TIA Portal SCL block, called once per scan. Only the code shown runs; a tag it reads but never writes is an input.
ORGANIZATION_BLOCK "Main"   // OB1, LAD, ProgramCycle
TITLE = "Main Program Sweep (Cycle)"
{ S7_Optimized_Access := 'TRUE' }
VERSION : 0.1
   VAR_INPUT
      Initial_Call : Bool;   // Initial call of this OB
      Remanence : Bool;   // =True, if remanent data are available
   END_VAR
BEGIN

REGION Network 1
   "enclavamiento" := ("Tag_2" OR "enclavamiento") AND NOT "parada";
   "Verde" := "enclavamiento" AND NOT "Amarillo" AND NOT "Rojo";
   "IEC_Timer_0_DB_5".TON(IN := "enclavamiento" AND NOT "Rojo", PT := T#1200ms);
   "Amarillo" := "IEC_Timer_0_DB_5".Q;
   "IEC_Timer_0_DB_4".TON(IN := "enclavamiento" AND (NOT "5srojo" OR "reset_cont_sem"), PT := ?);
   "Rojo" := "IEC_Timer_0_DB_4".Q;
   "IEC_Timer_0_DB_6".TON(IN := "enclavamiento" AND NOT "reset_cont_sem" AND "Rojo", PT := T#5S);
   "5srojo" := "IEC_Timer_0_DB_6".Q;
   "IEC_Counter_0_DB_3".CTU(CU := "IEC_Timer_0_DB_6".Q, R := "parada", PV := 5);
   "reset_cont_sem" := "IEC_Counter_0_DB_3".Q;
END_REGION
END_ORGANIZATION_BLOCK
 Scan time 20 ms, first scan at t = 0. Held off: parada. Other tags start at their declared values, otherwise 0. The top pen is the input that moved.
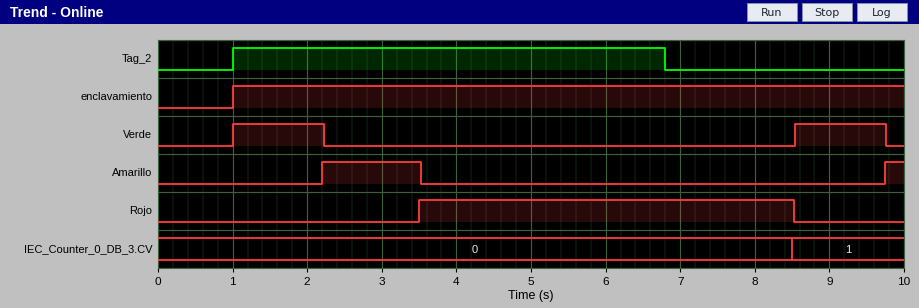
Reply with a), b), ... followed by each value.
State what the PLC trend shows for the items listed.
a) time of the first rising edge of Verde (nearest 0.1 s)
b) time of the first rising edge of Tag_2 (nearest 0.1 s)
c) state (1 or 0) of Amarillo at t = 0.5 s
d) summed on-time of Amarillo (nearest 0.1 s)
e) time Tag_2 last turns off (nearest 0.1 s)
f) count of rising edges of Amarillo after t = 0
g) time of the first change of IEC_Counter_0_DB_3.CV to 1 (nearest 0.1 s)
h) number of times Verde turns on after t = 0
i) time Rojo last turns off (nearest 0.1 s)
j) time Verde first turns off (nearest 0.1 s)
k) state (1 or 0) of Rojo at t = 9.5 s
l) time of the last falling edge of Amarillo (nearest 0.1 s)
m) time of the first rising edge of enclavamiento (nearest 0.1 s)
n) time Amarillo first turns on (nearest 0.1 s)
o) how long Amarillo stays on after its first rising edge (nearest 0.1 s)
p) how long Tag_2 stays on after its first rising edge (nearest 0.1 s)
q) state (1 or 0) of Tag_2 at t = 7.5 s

a) 1.0 s
b) 1.0 s
c) 0
d) 1.6 s
e) 6.8 s
f) 2
g) 8.5 s
h) 2
i) 8.5 s
j) 2.2 s
k) 0
l) 3.5 s
m) 1.0 s
n) 2.2 s
o) 1.3 s
p) 5.8 s
q) 0
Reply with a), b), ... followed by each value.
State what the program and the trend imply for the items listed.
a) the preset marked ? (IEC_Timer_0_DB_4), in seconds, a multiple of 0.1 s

a) 2.5 s
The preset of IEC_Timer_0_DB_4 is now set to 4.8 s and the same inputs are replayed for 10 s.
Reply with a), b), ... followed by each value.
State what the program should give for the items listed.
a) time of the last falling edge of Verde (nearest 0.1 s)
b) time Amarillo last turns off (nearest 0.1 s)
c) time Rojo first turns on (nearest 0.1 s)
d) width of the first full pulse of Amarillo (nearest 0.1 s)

a) 2.2 s
b) 5.8 s
c) 5.8 s
d) 3.6 s
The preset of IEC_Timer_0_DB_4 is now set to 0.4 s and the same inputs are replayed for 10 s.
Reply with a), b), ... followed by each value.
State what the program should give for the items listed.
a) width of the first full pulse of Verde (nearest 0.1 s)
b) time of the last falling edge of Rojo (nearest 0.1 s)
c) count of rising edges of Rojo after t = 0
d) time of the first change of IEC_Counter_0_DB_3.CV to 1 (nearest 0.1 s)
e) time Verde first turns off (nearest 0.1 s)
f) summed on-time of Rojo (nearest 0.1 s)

a) 0.4 s
b) 6.4 s
c) 2
d) 6.4 s
e) 1.4 s
f) 8.2 s
